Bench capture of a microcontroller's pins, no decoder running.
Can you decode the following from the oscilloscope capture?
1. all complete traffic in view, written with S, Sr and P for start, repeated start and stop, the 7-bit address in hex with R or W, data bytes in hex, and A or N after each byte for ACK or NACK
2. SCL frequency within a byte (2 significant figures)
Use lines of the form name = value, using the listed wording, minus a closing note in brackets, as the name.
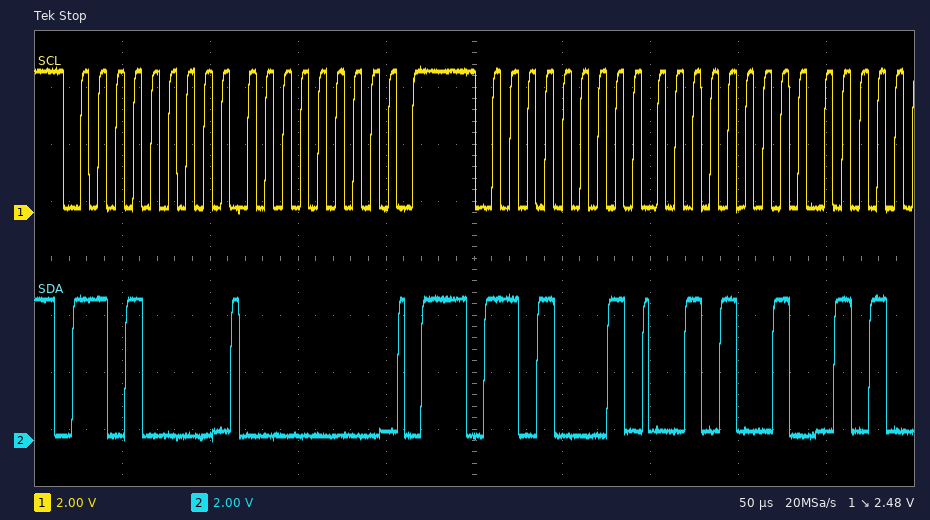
all complete traffic in view, written with S, Sr and P for start, repeated start and stop, the 7-bit address in hex with R or W, data bytes in hex, and A or N after each byte for ACK or NACK = S 68W A 00 A P S 68R A 29 A
SCL frequency within a byte = 100 kHz
